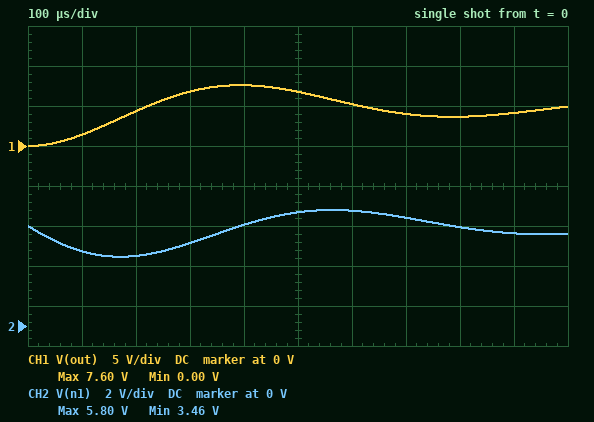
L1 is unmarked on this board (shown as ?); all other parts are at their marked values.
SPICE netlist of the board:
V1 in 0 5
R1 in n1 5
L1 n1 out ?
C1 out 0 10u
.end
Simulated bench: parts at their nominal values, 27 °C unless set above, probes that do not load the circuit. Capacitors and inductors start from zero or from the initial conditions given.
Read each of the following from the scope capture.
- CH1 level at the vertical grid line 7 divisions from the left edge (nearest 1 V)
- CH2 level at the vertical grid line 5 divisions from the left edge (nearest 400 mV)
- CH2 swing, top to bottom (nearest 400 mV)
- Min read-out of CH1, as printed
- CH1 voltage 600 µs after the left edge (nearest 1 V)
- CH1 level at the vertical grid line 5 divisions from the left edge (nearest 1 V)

4 V
5.6 V
2.4 V
0.00 V
5 V
7 V
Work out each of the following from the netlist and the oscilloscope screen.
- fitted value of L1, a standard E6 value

1.5 mH
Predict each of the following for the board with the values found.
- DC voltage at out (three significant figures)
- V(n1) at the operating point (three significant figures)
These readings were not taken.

5.00 V
5.00 V
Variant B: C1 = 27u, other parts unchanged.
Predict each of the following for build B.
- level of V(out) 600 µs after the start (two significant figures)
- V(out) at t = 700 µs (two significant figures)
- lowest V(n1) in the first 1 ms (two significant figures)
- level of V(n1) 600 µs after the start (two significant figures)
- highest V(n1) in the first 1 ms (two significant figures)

6.5 V
6.6 V
2.8 V
4.6 V
5.7 V
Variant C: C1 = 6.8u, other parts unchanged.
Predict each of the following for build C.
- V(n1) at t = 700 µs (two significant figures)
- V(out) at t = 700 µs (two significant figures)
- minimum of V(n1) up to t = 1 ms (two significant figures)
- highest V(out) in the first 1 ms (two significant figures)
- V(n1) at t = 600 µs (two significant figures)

4.7 V
3.5 V
3.7 V
7.9 V
5.3 V
